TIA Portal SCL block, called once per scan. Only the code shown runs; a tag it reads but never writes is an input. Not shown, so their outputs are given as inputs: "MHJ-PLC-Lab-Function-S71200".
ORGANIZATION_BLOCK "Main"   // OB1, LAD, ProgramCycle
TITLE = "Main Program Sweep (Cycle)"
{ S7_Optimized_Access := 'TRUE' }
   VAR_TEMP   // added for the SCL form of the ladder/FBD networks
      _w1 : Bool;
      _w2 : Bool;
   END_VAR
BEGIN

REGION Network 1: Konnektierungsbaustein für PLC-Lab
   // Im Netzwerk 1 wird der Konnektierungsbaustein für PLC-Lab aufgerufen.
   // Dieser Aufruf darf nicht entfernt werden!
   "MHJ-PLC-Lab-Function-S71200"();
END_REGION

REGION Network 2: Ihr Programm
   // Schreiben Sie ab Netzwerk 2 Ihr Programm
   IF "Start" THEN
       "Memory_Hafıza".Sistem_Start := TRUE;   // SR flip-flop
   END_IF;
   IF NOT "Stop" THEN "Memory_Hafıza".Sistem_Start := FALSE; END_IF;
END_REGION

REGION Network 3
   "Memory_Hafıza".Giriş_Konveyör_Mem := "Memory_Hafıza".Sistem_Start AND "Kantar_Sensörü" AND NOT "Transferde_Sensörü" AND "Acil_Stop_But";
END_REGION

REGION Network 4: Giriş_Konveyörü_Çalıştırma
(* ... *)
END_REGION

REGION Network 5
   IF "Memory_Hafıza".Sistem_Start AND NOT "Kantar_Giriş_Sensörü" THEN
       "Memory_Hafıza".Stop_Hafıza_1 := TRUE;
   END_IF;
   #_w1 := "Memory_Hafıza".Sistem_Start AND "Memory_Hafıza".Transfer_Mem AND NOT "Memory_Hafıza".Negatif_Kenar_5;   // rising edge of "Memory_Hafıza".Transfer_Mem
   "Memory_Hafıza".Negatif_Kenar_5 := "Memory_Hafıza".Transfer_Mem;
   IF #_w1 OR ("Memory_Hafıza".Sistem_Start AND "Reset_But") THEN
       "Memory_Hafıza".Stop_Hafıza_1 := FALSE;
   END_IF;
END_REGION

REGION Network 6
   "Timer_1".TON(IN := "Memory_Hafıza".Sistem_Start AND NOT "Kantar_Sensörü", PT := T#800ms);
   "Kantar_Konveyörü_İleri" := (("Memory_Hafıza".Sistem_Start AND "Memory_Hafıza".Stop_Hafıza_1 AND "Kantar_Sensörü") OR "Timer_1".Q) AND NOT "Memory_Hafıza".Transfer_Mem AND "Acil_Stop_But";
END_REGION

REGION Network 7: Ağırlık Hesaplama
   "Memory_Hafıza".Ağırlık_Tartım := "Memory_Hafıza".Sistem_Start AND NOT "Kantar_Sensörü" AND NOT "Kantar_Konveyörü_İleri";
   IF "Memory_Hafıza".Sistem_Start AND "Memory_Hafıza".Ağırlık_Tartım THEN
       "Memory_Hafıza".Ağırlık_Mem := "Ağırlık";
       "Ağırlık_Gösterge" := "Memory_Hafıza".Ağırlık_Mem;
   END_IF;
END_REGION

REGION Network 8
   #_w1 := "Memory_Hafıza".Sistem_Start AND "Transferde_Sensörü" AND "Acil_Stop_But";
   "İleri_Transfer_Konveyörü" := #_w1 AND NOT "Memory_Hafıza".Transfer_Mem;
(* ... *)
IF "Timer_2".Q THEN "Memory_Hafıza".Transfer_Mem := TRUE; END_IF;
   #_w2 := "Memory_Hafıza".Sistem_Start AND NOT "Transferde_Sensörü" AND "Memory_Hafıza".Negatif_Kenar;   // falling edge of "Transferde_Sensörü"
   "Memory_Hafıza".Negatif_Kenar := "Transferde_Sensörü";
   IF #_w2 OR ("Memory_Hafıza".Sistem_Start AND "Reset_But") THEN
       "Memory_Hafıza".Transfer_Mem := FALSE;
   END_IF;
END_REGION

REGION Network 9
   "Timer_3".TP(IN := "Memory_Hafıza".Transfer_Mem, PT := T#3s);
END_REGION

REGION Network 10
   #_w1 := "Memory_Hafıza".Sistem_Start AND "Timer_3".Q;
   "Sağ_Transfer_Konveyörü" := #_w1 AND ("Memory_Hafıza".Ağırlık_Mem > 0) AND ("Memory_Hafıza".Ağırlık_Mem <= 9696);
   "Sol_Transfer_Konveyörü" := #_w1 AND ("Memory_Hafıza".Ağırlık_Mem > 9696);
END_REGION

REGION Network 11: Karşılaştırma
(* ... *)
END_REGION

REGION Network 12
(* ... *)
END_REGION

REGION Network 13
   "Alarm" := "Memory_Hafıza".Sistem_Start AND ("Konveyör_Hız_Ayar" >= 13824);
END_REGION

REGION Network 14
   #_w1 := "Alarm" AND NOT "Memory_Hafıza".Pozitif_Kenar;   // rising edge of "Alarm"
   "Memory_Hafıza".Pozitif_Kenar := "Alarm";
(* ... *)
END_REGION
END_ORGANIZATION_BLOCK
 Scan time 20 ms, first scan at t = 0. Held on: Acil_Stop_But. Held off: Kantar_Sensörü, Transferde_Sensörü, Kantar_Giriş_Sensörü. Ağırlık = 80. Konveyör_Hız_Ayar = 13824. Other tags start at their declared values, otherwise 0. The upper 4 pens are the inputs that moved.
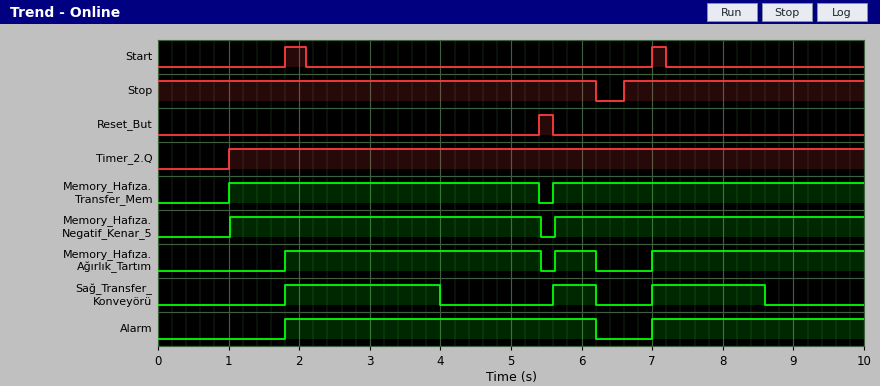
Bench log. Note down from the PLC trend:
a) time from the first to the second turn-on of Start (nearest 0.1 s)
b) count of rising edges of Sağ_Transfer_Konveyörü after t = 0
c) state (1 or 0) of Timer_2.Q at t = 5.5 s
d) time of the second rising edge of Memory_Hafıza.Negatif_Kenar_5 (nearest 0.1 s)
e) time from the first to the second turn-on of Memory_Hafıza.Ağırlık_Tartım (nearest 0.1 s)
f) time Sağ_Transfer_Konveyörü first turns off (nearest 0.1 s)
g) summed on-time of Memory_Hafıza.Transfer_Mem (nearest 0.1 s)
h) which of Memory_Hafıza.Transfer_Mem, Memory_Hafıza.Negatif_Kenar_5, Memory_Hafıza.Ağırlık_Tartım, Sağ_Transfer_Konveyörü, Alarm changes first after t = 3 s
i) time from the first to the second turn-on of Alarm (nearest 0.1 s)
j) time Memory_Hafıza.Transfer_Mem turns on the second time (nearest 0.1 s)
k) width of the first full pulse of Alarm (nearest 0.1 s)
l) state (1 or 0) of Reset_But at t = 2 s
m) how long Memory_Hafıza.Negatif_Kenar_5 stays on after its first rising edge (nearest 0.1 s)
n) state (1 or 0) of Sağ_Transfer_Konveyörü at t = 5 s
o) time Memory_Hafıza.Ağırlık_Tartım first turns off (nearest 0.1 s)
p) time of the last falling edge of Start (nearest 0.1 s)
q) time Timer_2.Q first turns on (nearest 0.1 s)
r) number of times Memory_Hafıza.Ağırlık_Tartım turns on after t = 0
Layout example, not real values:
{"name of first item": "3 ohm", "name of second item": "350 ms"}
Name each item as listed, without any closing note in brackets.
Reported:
{"time from the first to the second turn-on of Start": "5.2 s", "count of rising edges of Sağ_Transfer_Konveyörü after t = 0": "3", "state (1 or 0) of Timer_2.Q at t = 5.5 s": "1", "time of the second rising edge of Memory_Hafıza.Negatif_Kenar_5": "5.6 s", "time from the first to the second turn-on of Memory_Hafıza.Ağırlık_Tartım": "3.8 s", "time Sağ_Transfer_Konveyörü first turns off": "4.0 s", "summed on-time of Memory_Hafıza.Transfer_Mem": "8.8 s", "which of Memory_Hafıza.Transfer_Mem, Memory_Hafıza.Negatif_Kenar_5, Memory_Hafıza.Ağırlık_Tartım, Sağ_Transfer_Konveyörü, Alarm changes first after t = 3 s": "Sağ_Transfer_Konveyörü", "time from the first to the second turn-on of Alarm": "5.2 s", "time Memory_Hafıza.Transfer_Mem turns on the second time": "5.6 s", "width of the first full pulse of Alarm": "4.4 s", "state (1 or 0) of Reset_But at t = 2 s": "0", "how long Memory_Hafıza.Negatif_Kenar_5 stays on after its first rising edge": "4.4 s", "state (1 or 0) of Sağ_Transfer_Konveyörü at t = 5 s": "0", "time Memory_Hafıza.Ağırlık_Tartım first turns off": "5.4 s", "time of the last falling edge of Start": "7.2 s", "time Timer_2.Q first turns on": "1.0 s", "number of times Memory_Hafıza.Ağırlık_Tartım turns on after t = 0": "3"}
